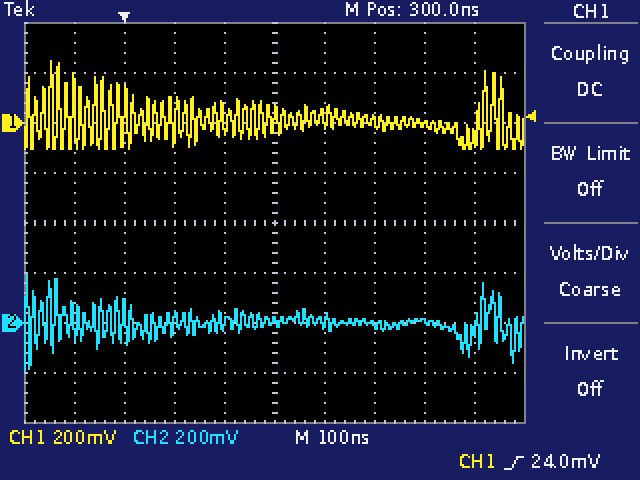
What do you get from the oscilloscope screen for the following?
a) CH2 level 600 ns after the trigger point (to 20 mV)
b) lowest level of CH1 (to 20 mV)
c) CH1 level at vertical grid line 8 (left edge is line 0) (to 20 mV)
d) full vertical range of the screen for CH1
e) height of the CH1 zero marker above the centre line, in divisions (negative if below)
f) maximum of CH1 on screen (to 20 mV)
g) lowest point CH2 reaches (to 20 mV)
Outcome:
0 mV
-100 mV
0 mV
1.6 V
+2.0 div
240 mV
-200 mV
